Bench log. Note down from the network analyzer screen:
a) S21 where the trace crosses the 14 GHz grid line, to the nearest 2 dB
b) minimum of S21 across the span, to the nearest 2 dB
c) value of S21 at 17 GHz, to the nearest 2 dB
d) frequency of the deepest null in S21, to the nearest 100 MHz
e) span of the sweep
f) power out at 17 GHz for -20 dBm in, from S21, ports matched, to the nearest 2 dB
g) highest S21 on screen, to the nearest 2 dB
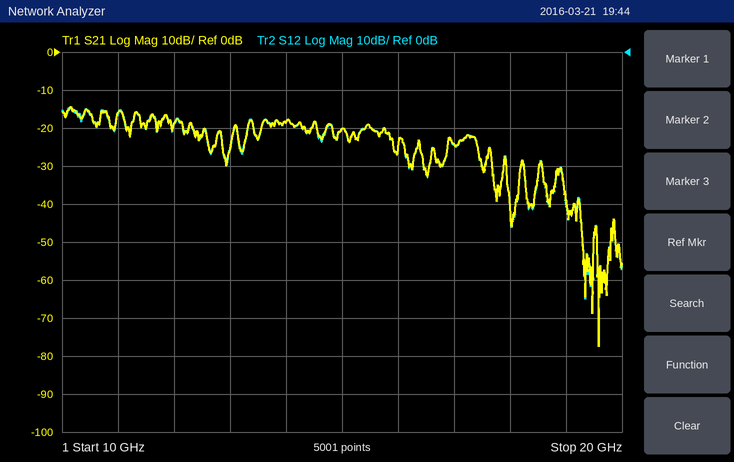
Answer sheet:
-18 dB
-78 dB
-24 dB
19.6 GHz
10 GHz
-44 dBm
-14 dB
